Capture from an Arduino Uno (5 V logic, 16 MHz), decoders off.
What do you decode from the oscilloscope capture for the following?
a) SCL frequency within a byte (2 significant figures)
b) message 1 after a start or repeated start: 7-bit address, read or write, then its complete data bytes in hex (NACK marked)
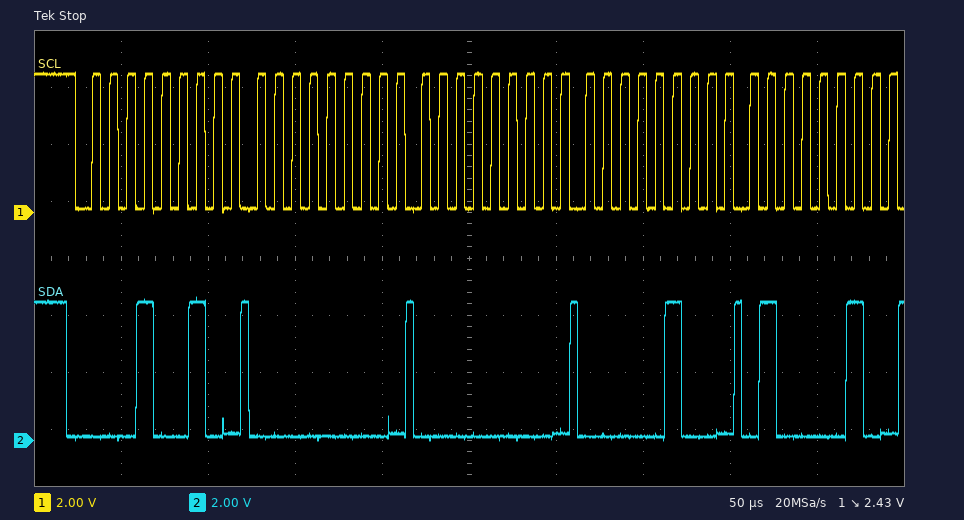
100 kHz
0x09 write: 00 00 04 42
